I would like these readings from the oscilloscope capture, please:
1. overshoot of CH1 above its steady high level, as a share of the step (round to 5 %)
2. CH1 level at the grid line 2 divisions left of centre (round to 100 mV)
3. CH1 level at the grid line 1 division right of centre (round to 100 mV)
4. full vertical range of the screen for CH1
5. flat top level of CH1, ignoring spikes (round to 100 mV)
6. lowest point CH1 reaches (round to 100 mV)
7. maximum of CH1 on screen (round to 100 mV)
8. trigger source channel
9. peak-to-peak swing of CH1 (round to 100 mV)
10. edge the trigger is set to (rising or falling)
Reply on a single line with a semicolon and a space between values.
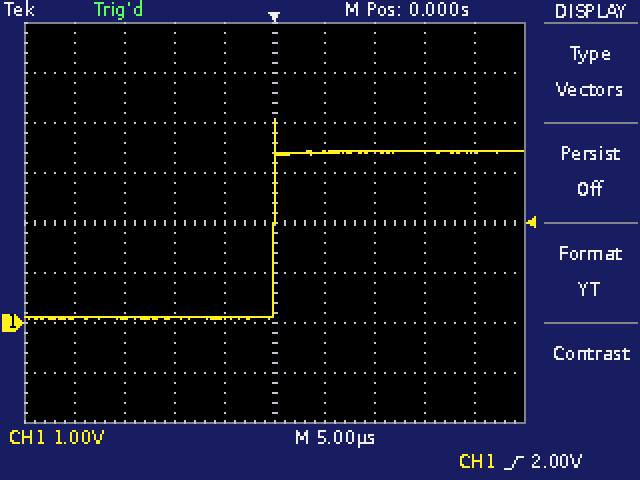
20 %; 100 mV; 3.4 V; 8 V; 3.4 V; 100 mV; 4.1 V; CH1; 4.0 V; rising
